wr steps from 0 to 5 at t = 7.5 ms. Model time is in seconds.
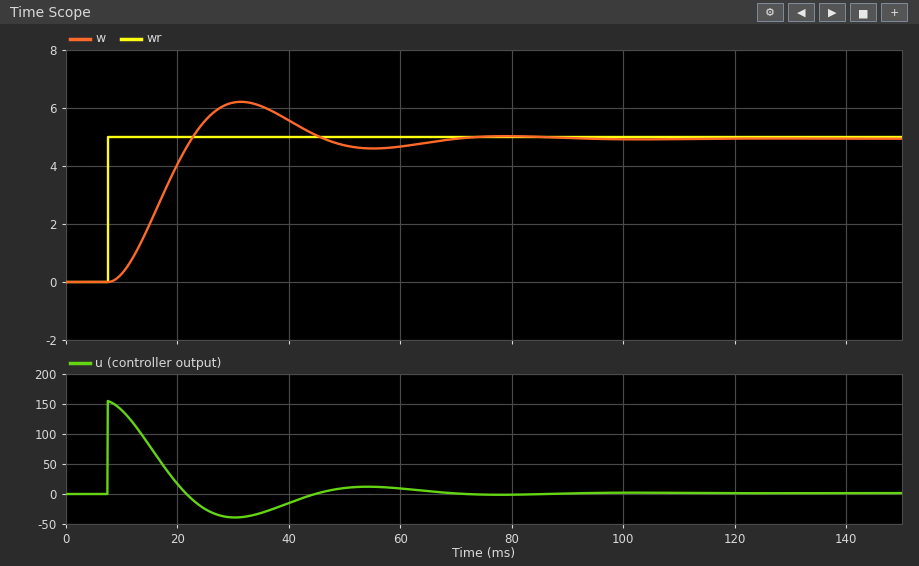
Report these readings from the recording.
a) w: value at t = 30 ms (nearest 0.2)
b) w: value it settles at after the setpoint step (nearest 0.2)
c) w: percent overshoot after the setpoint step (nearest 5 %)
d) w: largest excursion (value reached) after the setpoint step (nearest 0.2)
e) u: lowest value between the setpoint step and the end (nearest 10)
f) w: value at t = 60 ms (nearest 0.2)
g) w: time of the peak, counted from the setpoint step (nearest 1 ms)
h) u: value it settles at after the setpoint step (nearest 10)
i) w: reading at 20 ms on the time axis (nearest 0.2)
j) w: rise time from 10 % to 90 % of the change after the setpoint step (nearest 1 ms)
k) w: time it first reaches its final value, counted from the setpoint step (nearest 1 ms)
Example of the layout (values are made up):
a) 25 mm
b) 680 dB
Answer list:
a) 6.2
b) 5.0
c) 25 %
d) 6.2
e) -40
f) 4.6
g) 24 ms
h) 0
i) 4.0
j) 10 ms
k) 15 ms
